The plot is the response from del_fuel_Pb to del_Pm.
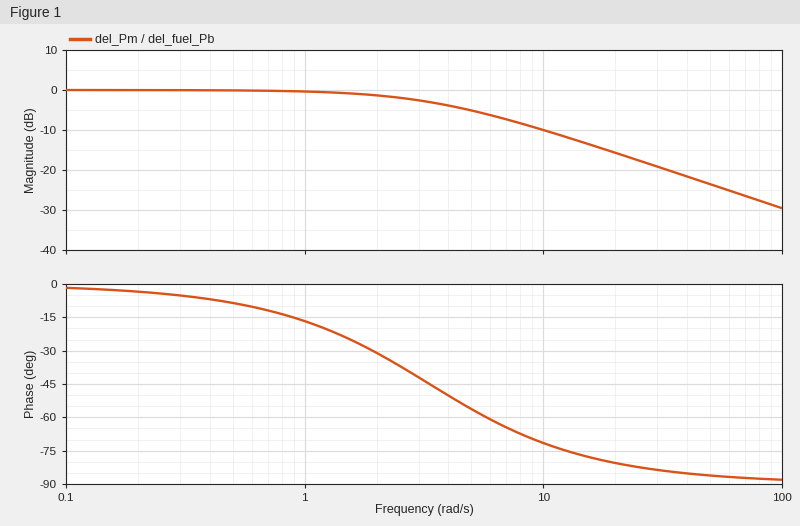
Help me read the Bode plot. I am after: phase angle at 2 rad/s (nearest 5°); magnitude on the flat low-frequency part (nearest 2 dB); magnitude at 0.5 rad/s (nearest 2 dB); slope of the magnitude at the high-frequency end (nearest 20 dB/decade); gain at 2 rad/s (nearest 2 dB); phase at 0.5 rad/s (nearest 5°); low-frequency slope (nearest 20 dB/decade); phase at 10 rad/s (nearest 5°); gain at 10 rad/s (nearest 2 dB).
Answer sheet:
-30°
0 dB
0 dB
-20 dB/decade
-2 dB
-10°
0 dB/decade
-70°
-10 dB
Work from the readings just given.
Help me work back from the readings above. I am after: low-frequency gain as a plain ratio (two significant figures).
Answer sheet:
1.0
